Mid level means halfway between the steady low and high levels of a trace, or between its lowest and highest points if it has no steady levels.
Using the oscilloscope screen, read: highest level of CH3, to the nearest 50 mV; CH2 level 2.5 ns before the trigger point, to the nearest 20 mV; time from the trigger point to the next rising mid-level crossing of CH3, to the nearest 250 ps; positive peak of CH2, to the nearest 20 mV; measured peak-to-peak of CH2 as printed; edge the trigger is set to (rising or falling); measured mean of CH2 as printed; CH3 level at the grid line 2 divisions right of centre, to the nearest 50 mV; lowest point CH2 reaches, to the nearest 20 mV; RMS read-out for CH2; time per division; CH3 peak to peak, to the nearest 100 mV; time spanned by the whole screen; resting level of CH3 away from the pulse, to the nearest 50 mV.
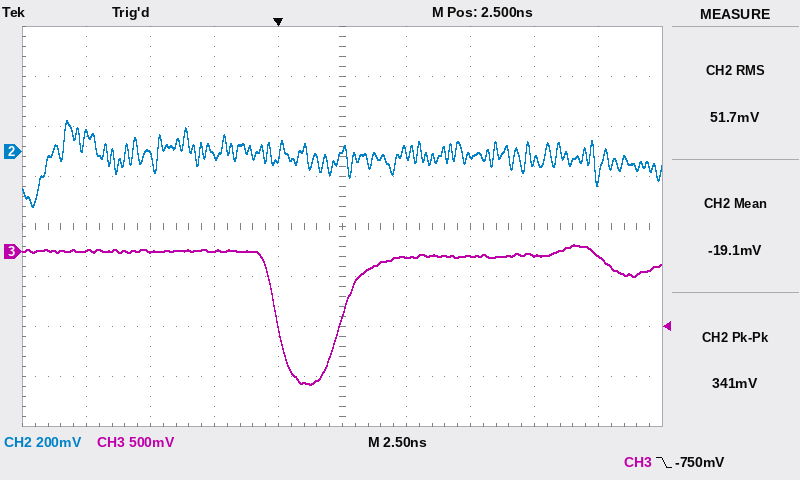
50 mV
-20 mV
2.50 ns
120 mV
341 mV
falling
-19.1 mV
-50 mV
-220 mV
51.7 mV
2.5 ns
1.40 V
25 ns
0 mV
